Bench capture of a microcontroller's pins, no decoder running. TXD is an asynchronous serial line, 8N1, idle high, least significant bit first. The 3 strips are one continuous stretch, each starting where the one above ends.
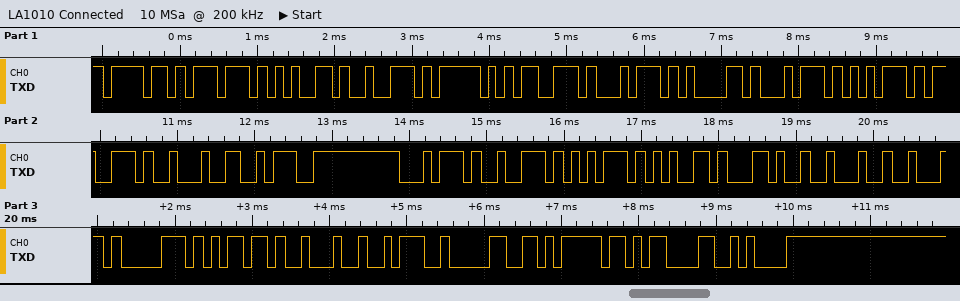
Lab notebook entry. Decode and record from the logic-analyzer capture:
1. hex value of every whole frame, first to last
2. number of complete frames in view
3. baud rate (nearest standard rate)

6F 77 65 72 5F 73 74 61 74 75 73 22 3A 74 72 75 65 2C 22 62 70 6D 22 3A 30 7D 0D 0A
28
9600 baud
